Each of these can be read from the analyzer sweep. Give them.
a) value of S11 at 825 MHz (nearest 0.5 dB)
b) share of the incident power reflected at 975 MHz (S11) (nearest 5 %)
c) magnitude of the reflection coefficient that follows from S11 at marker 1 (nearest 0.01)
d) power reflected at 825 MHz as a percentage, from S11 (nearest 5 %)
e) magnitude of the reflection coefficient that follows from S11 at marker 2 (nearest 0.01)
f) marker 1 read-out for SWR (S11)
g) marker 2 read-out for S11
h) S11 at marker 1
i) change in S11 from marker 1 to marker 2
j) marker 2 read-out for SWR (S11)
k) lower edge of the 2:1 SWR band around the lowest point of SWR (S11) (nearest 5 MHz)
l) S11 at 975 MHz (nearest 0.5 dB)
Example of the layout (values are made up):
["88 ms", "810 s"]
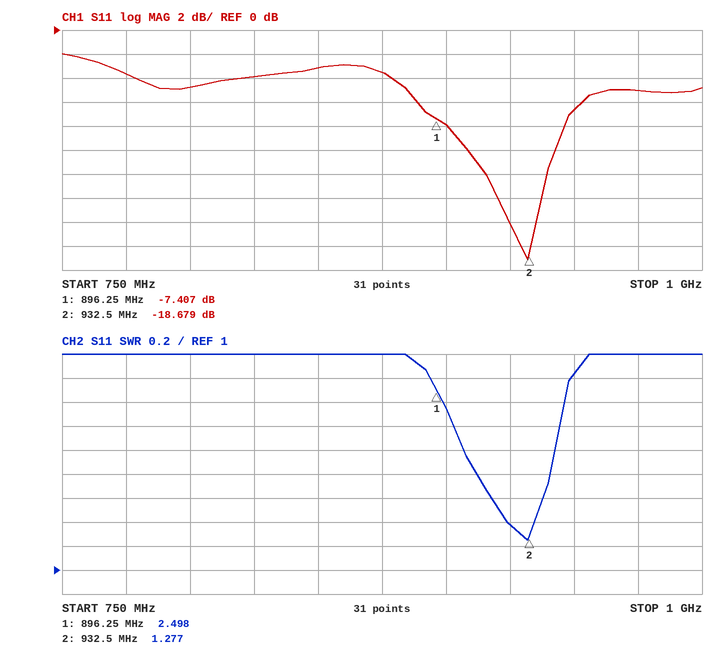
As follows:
["-4.0 dB", "30 %", "0.43", "40 %", "0.12", "2.498", "-18.679 dB", "-7.407 dB", "-11.272 dB", "1.277", "905 MHz", "-5.0 dB"]
